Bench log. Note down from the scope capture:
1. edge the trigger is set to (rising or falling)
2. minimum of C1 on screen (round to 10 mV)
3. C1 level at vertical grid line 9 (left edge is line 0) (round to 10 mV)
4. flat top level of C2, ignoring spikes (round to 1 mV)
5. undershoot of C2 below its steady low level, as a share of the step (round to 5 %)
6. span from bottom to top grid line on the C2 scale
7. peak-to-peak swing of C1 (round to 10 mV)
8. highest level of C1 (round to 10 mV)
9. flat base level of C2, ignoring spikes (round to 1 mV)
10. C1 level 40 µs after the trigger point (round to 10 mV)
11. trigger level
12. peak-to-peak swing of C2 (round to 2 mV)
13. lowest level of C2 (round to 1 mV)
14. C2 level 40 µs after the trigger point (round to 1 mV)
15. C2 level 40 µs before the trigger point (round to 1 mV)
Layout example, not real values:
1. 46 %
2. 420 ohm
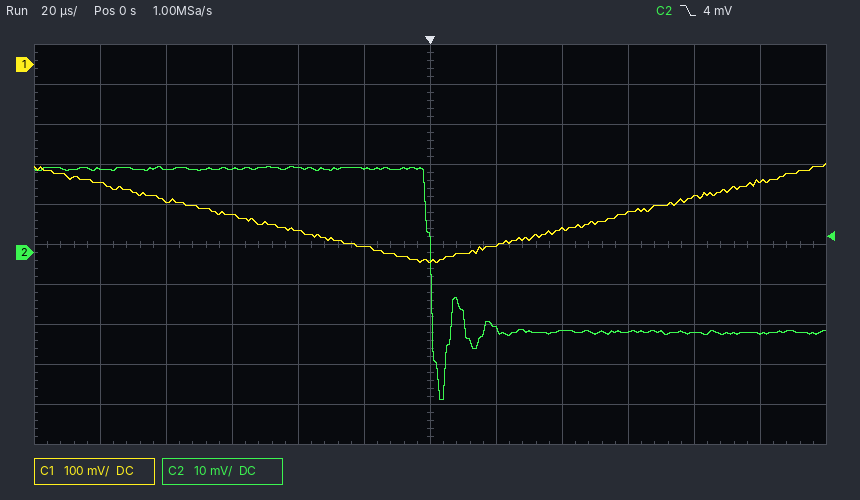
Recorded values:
1. falling
2. -500 mV
3. -370 mV
4. 21 mV
5. 40 %
6. 100 mV
7. 250 mV
8. -250 mV
9. -20 mV
10. -410 mV
11. 4 mV
12. 58 mV
13. -37 mV
14. -20 mV
15. 21 mV
